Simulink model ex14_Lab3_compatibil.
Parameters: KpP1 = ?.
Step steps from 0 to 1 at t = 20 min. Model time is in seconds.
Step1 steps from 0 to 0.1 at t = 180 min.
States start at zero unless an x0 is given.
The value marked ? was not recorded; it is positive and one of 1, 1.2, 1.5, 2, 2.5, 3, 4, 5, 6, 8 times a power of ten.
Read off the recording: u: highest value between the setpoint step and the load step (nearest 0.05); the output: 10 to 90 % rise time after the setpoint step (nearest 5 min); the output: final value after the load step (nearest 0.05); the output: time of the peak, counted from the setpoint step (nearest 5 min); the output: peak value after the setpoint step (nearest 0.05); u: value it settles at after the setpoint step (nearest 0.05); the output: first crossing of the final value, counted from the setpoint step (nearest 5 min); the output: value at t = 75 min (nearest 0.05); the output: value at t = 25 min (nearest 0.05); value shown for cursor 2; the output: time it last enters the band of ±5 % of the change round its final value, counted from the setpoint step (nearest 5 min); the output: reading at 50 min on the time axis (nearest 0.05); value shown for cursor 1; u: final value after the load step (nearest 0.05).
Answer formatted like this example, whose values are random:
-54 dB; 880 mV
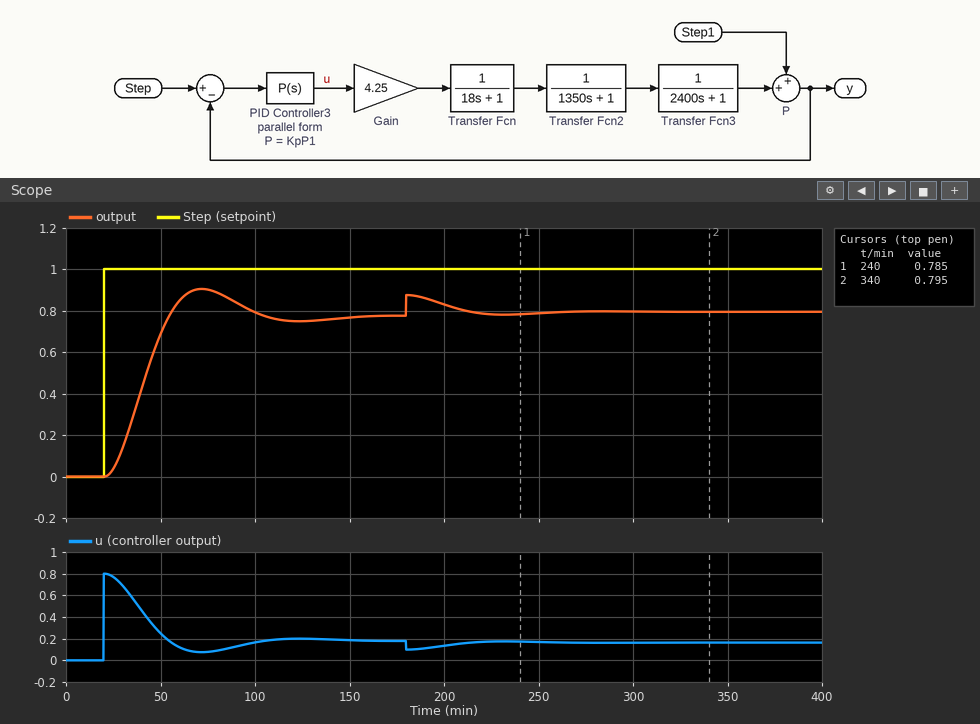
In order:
0.80; 25 min; 0.80; 50 min; 0.90; 0.20; 35 min; 0.90; 0.05; 0.795; 75 min; 0.70; 0.785; 0.15
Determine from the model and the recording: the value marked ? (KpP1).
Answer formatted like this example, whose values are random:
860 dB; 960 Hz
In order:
0.8
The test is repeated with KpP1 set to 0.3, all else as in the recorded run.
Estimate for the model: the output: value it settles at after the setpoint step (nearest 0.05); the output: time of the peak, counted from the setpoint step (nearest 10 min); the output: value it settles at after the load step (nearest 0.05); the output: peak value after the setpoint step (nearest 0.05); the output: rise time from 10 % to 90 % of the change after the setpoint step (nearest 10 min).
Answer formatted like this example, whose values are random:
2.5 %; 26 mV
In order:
0.55; 90 min; 0.60; 0.60; 40 min
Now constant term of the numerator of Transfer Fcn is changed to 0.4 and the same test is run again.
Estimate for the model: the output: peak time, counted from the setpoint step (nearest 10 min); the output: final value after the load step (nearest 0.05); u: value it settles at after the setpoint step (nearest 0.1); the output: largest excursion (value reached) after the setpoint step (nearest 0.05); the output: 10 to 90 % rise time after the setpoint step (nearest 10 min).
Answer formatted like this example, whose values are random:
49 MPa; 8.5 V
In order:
80 min; 0.60; 0.3; 0.60; 40 min
